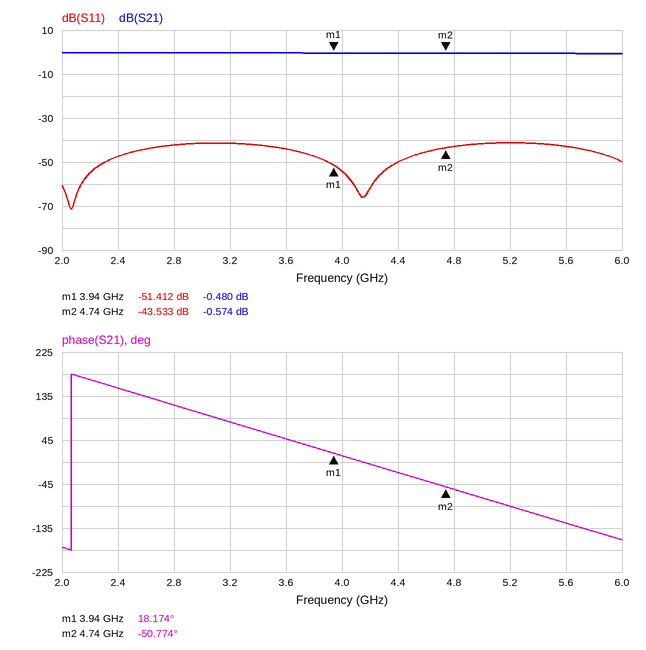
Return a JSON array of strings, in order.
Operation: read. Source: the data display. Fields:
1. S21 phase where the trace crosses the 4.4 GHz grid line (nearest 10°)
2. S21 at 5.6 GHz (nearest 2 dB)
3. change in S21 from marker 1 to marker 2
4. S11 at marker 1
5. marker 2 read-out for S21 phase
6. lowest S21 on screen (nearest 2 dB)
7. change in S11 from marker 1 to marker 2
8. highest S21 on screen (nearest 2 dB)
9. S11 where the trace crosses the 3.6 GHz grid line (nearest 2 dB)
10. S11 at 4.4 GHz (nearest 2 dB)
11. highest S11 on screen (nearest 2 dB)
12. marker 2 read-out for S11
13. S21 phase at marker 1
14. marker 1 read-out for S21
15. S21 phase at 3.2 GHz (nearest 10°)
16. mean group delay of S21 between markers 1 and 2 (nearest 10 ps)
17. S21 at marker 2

["-20°", "0 dB", "-0.094 dB", "-51.412 dB", "-50.774°", "0 dB", "7.879 dB", "0 dB", "-44 dB", "-50 dB", "-42 dB", "-43.533 dB", "18.174°", "-0.480 dB", "80°", "240 ps", "-0.574 dB"]
